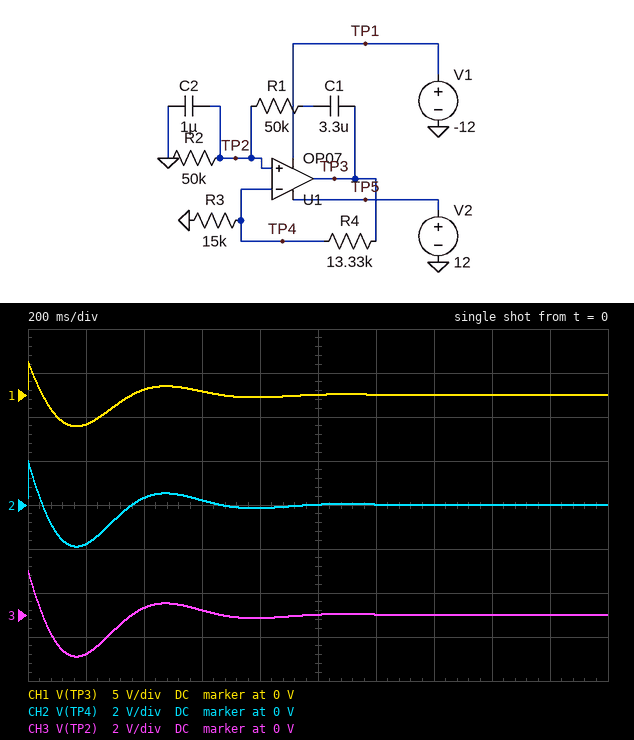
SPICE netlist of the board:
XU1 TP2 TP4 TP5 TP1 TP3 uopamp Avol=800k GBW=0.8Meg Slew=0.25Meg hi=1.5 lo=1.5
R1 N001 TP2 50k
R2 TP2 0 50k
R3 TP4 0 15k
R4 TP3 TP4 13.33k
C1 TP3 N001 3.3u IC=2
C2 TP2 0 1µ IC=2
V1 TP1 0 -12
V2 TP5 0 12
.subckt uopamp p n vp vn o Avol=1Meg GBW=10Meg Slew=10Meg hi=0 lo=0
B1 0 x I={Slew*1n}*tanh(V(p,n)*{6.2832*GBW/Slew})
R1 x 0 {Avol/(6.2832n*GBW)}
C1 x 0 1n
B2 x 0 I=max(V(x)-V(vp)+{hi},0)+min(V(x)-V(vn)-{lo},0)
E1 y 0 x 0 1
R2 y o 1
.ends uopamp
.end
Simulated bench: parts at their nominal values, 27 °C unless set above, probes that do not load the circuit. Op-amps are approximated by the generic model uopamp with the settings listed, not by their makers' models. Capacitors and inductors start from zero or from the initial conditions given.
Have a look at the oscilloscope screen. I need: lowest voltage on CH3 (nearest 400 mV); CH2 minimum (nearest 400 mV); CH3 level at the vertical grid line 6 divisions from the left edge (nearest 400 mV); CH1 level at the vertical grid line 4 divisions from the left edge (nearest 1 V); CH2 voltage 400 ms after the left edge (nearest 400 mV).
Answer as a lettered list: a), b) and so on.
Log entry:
a) -2.0 V
b) -2.0 V
c) 0 V
d) 0 V
e) 400 mV
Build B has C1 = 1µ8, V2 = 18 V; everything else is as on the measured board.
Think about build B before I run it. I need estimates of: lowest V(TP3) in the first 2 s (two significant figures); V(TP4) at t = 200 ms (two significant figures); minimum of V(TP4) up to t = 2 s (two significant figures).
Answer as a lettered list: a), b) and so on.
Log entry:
a) -2.1 V
b) -750 mV
c) -1.1 V
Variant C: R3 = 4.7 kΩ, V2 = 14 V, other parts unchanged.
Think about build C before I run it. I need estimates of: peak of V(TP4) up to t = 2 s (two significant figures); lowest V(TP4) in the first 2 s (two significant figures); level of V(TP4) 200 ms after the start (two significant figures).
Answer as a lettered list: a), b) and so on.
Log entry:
a) 3.3 V
b) -2.7 V
c) 3.0 V
